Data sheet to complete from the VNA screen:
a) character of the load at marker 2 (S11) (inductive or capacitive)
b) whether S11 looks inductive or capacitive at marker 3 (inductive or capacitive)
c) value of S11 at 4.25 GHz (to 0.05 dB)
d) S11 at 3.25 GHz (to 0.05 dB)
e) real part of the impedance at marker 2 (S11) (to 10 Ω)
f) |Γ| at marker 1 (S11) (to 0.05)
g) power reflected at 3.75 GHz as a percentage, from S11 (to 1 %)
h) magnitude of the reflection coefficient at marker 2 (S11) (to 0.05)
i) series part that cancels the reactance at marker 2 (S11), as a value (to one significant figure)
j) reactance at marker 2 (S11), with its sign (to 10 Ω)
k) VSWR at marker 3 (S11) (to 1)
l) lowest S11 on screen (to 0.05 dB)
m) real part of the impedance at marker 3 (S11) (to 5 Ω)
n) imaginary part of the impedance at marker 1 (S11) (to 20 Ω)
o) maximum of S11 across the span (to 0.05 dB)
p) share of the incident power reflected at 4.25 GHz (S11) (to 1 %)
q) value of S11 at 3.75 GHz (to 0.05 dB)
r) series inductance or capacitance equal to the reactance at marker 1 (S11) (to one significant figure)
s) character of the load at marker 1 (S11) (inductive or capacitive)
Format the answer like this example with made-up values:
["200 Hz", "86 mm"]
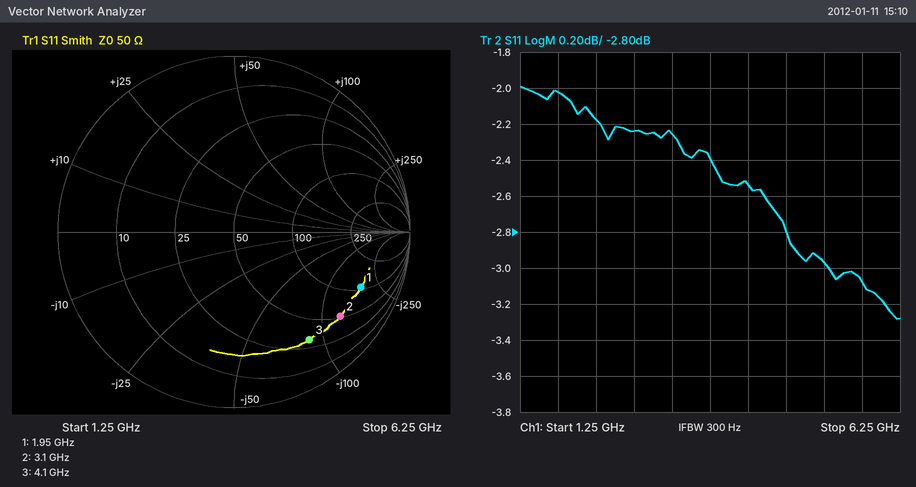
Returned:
["capacitive", "capacitive", "-2.55 dB", "-2.25 dB", "50 Ω", "0.80", "58 %", "0.75", "6 nH", "-120 Ω", "7", "-3.30 dB", "30 Ω", "-180 Ω", "-2.00 dB", "56 %", "-2.40 dB", "500 fF", "capacitive"]
